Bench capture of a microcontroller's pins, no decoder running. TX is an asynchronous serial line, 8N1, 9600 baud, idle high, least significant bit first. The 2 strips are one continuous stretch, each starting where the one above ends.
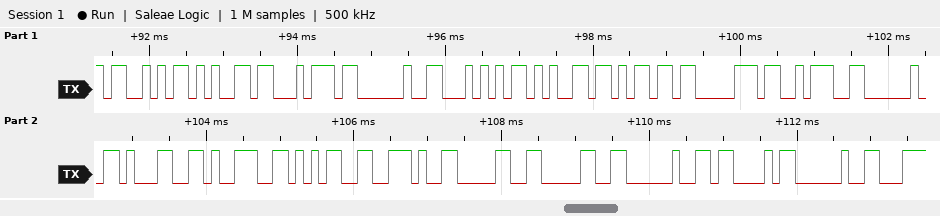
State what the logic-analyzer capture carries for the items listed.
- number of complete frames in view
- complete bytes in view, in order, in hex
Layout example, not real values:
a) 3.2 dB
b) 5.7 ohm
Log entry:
a) 19
b) 53 65 74 20 54 65 6D 70 3A 20 31 39 35 2E 30 30 20 43 20
